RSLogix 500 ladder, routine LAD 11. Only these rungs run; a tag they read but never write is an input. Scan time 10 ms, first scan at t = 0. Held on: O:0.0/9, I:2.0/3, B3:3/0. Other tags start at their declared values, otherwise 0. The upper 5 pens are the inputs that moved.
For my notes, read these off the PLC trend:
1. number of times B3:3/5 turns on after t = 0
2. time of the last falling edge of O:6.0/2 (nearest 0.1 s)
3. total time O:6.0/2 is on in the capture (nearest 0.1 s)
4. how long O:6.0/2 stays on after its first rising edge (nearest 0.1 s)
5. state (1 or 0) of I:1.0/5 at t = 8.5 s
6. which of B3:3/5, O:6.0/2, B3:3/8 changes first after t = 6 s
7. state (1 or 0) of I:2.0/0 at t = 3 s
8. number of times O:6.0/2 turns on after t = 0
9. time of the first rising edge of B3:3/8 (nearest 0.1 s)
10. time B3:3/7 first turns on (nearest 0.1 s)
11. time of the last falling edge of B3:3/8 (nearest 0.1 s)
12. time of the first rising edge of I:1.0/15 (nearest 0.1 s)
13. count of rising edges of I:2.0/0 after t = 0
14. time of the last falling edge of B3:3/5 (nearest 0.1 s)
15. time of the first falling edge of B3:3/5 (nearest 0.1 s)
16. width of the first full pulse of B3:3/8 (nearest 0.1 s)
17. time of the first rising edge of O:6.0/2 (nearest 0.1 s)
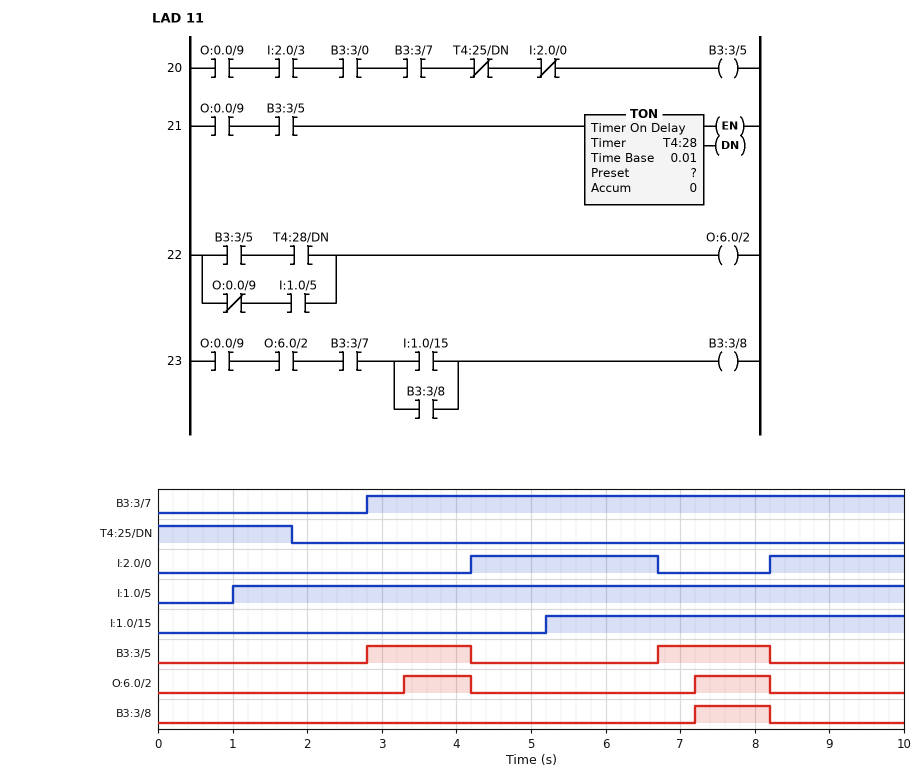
2
8.2 s
1.9 s
0.9 s
1
B3:3/5
0
2
7.2 s
2.8 s
8.2 s
5.2 s
2
8.2 s
4.2 s
1.0 s
3.3 s
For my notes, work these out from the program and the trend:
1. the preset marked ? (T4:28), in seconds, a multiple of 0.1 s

0.5 s
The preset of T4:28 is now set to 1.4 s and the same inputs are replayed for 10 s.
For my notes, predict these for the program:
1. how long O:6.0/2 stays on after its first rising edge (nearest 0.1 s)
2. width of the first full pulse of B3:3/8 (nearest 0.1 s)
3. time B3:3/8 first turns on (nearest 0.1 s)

0.1 s
0.1 s
8.1 s
